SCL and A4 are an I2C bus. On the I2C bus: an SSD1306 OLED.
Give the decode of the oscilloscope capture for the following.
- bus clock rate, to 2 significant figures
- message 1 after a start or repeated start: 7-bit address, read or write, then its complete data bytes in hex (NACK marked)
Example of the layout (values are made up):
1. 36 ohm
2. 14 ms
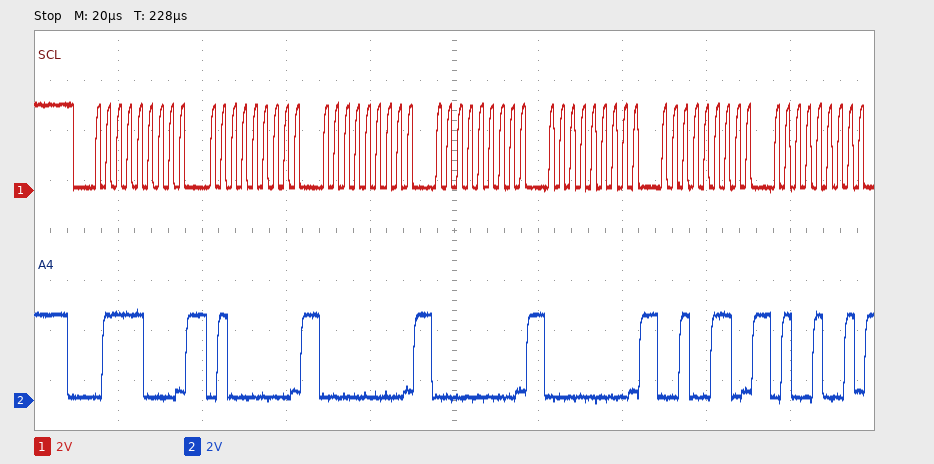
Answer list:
1. 400 kHz
2. 0x3C write: 40 00 00 00 26 49
